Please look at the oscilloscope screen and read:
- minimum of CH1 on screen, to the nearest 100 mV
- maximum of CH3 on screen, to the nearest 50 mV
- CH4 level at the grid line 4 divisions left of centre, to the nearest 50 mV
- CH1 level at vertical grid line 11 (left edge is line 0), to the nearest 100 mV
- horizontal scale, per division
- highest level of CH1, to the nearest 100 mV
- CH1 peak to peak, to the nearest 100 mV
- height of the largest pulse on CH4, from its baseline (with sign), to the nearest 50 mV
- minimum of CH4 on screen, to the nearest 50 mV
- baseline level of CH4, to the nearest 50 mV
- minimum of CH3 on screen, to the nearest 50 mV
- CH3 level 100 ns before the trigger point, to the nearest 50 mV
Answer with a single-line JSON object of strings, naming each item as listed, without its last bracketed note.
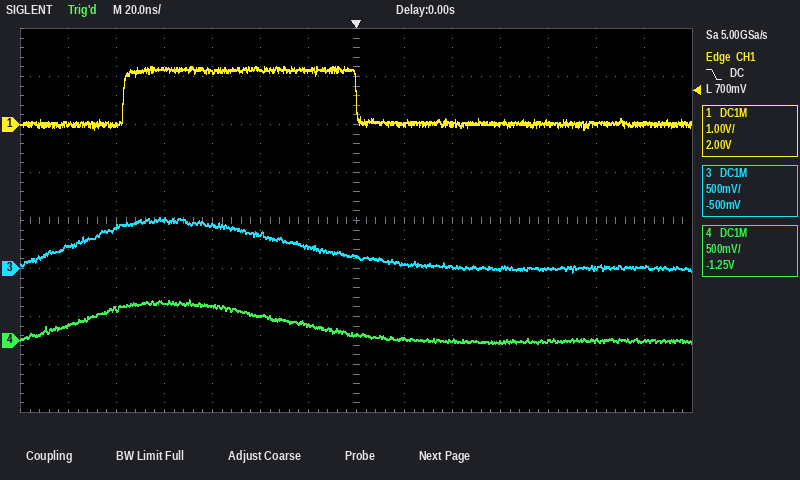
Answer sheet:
{"minimum of CH1 on screen, to the nearest 100 mV": "-100 mV", "maximum of CH3 on screen, to the nearest 50 mV": "550 mV", "CH4 level at the grid line 4 divisions left of centre, to the nearest 50 mV": "400 mV", "CH1 level at vertical grid line 11 (left edge is line 0), to the nearest 100 mV": "0.0 V", "horizontal scale, per division": "20 ns", "highest level of CH1, to the nearest 100 mV": "1.2 V", "CH1 peak to peak, to the nearest 100 mV": "1.3 V", "height of the largest pulse on CH4, from its baseline (with sign), to the nearest 50 mV": "+400 mV", "minimum of CH4 on screen, to the nearest 50 mV": "-50 mV", "baseline level of CH4, to the nearest 50 mV": "0 mV", "minimum of CH3 on screen, to the nearest 50 mV": "-50 mV", "CH3 level 100 ns before the trigger point, to the nearest 50 mV": "450 mV"}
